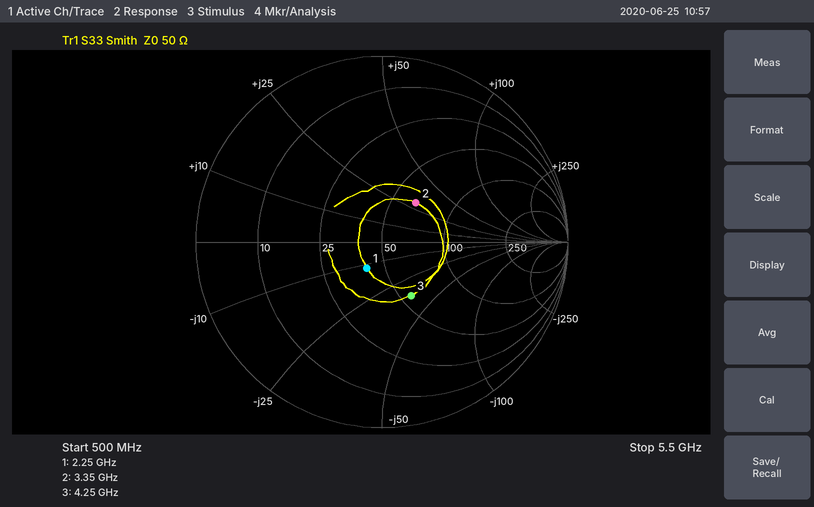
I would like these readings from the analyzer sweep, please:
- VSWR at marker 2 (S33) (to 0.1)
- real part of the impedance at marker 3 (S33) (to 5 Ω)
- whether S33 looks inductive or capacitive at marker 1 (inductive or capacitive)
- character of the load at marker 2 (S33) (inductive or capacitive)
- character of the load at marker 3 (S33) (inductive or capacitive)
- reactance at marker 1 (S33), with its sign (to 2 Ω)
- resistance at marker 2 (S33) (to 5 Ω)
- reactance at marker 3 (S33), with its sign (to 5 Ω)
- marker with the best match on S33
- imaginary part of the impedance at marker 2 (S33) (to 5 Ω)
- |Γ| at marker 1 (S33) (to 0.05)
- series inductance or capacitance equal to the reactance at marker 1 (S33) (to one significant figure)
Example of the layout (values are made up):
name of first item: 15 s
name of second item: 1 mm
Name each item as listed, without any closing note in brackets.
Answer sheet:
VSWR at marker 2 (S33): 1.8
real part of the impedance at marker 3 (S33): 55 Ω
whether S33 looks inductive or capacitive at marker 1: capacitive
character of the load at marker 2 (S33): inductive
character of the load at marker 3 (S33): capacitive
reactance at marker 1 (S33), with its sign: -12 Ω
resistance at marker 2 (S33): 65 Ω
reactance at marker 3 (S33), with its sign: -35 Ω
marker with the best match on S33: marker 1
imaginary part of the impedance at marker 2 (S33): +30 Ω
|Γ| at marker 1 (S33): 0.15
series inductance or capacitance equal to the reactance at marker 1 (S33): 6 pF
